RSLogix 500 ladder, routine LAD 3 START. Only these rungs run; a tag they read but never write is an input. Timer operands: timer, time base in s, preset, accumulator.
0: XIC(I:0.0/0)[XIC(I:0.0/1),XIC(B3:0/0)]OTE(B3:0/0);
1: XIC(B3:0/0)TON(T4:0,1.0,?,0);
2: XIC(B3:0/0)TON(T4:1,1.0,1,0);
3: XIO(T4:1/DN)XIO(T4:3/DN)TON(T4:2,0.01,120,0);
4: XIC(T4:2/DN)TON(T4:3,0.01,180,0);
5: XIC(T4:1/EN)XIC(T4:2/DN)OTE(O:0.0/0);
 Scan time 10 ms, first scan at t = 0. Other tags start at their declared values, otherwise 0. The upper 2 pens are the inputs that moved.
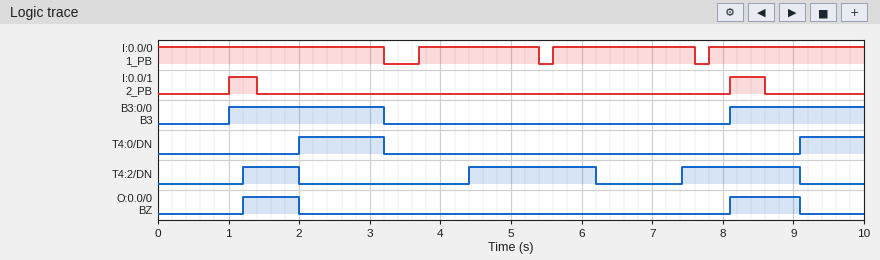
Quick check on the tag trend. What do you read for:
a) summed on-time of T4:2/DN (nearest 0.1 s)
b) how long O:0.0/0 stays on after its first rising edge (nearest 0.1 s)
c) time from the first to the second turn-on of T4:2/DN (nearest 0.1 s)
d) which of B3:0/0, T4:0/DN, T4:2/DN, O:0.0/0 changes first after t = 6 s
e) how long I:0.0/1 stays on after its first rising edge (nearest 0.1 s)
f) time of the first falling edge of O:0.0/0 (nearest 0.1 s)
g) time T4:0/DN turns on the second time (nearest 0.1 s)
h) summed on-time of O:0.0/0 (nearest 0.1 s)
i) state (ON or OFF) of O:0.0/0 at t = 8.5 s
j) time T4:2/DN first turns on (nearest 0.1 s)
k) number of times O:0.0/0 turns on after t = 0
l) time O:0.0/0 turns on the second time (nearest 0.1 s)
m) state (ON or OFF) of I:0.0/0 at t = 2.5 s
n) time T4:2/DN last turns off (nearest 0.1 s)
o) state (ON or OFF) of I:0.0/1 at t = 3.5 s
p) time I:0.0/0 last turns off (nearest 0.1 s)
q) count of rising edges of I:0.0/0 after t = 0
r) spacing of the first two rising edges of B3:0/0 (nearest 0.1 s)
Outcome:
4.3 s
0.8 s
3.2 s
T4:2/DN
0.4 s
2.0 s
9.1 s
1.8 s
ON
1.2 s
2
8.1 s
ON
9.1 s
OFF
7.6 s
3
7.1 s
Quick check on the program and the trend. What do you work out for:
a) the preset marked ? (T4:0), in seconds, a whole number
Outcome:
1 s
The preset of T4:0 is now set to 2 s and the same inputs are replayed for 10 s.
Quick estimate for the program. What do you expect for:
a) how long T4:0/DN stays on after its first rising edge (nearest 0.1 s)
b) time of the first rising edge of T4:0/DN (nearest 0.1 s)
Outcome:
0.2 s
3.0 s
